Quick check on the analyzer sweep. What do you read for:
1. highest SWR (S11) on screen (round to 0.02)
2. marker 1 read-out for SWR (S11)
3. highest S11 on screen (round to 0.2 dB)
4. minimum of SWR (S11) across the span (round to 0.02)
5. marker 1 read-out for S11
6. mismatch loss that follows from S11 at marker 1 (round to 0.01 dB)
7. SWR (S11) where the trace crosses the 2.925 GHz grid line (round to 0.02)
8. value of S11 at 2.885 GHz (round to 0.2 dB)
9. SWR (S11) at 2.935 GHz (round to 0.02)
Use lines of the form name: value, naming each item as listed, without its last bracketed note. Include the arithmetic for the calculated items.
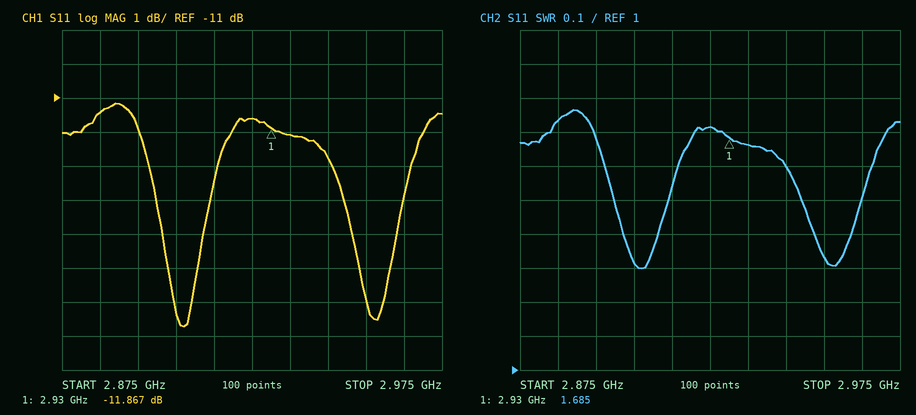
highest SWR (S11) on screen: 1.76
marker 1 read-out for SWR: 1.685
highest S11 on screen: -11.2 dB
minimum of SWR (S11) across the span: 1.30
marker 1 read-out for S11: -11.867 dB
mismatch loss that follows from S11 at marker 1: −10 log10(1 − 10^(-11.867/10)) ≈ 0.29 dB
SWR (S11) where the trace crosses the 2.925 GHz grid line: 1.72
value of S11 at 2.885 GHz: -11.4 dB
SWR (S11) at 2.935 GHz: 1.66
